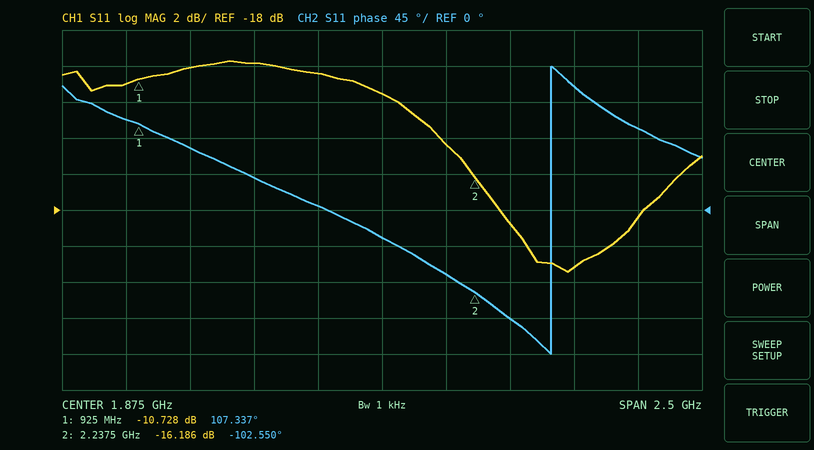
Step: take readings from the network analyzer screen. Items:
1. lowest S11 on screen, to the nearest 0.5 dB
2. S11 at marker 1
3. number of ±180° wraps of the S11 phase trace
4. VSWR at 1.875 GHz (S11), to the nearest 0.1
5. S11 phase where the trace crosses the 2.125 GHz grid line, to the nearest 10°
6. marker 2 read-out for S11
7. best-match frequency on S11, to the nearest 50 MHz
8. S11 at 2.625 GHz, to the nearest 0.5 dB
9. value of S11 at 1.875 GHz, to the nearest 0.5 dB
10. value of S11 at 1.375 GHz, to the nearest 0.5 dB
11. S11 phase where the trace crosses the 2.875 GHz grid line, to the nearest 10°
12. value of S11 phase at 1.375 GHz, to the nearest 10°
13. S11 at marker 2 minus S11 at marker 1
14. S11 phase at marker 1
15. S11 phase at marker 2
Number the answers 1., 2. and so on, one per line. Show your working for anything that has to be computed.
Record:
1. -21.5 dB
2. -10.728 dB
3. 1
4. |Γ| = 10^(-11.5/20) = 0.2661; VSWR = (1 + 0.2661)/(1 − 0.2661) ≈ 1.7
5. -80°
6. -16.186 dB
7. 2.60 GHz
8. -21.0 dB
9. -11.5 dB
10. -10.0 dB
11. 100°
12. 40°
13. -16.186 − (-10.728) = -5.458 dB
14. 107.337°
15. -102.550°
